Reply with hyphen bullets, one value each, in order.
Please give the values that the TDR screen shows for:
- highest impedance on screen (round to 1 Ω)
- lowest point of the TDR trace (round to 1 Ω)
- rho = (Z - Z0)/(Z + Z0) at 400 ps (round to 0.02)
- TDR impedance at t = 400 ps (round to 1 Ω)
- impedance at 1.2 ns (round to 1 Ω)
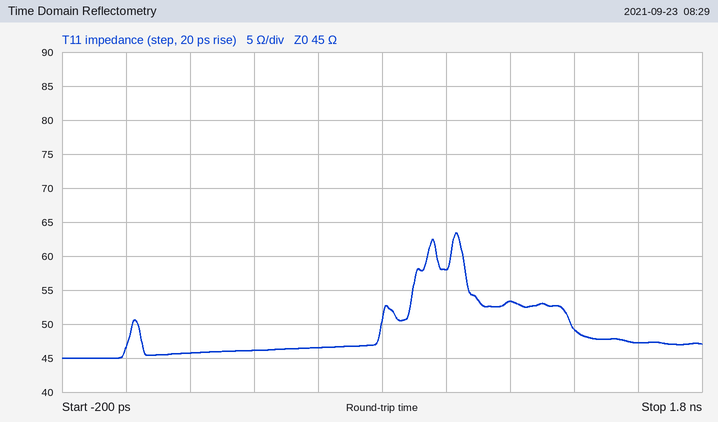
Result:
- 63 Ω
- 45 Ω
- +0.02
- 46 Ω
- 53 Ω
